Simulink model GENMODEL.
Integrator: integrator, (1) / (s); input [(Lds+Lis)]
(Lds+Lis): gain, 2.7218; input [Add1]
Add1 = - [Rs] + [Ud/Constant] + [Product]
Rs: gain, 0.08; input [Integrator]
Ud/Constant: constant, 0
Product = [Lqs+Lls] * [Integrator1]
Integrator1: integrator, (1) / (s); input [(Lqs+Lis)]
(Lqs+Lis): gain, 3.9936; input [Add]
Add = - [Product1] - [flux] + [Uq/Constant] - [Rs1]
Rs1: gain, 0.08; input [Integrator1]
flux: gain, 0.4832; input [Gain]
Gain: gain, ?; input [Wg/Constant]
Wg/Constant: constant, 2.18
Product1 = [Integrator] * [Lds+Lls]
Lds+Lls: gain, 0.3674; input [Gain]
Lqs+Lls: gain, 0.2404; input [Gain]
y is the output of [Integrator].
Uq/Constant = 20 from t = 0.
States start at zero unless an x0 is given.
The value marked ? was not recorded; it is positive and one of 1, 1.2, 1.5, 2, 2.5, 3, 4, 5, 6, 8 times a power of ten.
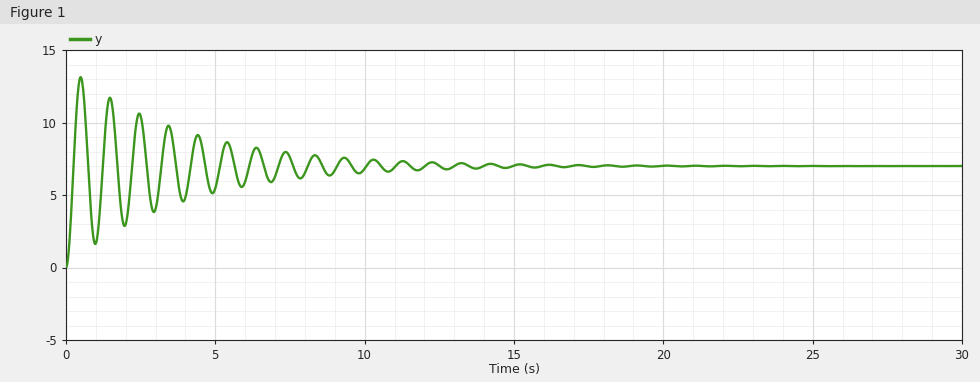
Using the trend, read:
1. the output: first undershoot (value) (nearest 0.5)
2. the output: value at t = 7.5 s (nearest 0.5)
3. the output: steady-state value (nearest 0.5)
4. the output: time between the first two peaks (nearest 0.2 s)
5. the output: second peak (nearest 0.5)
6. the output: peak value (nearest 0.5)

1.5
7.5
7.0
1.0 s
11.5
13.0
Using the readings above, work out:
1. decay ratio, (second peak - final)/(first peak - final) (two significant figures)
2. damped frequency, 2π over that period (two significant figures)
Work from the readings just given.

0.75
6.3 rad/s
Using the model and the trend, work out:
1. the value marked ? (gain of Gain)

3
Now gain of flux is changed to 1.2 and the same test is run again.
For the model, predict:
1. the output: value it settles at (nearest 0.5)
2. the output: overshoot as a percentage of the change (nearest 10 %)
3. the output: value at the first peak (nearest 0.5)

5.0
90 %
9.5
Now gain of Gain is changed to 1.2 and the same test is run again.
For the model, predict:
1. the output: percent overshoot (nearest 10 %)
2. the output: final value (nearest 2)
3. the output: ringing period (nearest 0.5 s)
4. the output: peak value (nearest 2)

70 %
20
2.5 s
34
